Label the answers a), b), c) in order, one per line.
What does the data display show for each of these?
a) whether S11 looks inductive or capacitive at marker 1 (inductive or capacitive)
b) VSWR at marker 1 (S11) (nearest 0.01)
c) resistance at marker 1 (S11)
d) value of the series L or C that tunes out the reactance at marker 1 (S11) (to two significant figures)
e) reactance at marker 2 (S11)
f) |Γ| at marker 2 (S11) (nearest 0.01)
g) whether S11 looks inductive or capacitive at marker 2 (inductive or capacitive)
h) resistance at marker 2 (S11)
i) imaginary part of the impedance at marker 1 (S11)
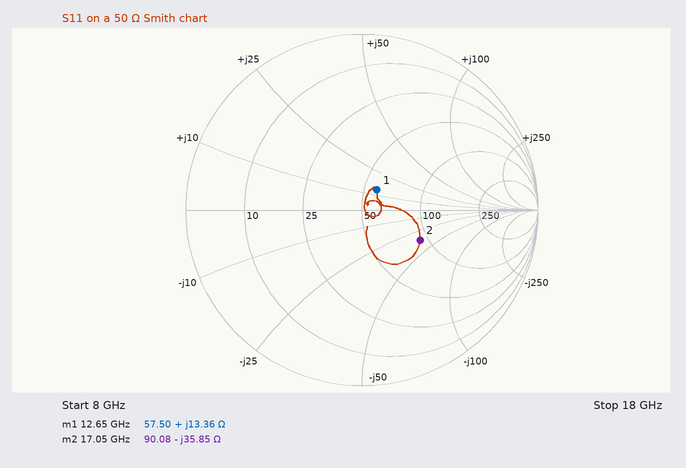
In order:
a) inductive
b) 1.33
c) 57.50 Ω
d) 940 fF
e) -35.85 Ω
f) 0.37
g) capacitive
h) 90.08 Ω
i) +13.36 Ω
